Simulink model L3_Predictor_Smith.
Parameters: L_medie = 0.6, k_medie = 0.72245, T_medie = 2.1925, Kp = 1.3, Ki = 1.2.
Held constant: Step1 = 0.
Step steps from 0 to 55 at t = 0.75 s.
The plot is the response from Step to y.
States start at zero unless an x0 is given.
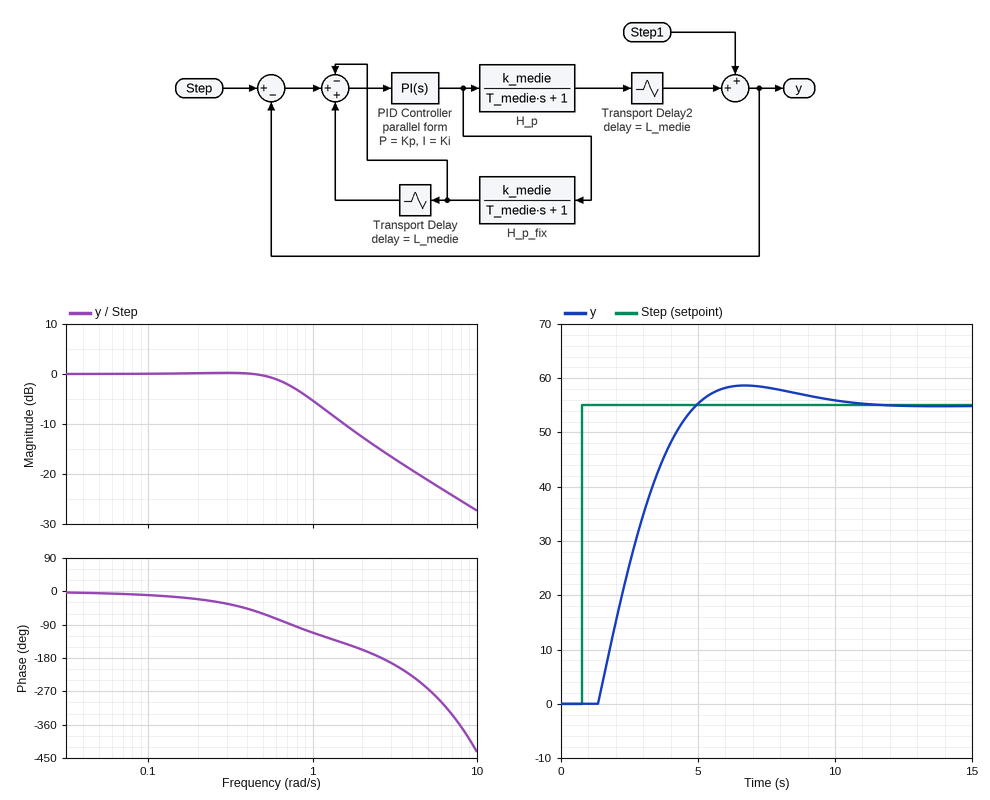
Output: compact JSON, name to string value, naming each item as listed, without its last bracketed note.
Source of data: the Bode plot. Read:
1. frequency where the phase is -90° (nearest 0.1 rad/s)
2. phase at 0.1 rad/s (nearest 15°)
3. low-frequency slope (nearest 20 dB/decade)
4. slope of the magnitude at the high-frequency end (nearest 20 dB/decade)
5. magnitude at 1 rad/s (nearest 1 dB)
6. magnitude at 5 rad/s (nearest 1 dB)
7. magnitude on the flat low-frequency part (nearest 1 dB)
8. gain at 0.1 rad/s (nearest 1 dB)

{"frequency where the phase is -90°": "0.7 rad/s", "phase at 0.1 rad/s": "-15°", "low-frequency slope": "0 dB/decade", "slope of the magnitude at the high-frequency end": "-20 dB/decade", "magnitude at 1 rad/s": "-5 dB", "magnitude at 5 rad/s": "-21 dB", "magnitude on the flat low-frequency part": "0 dB", "gain at 0.1 rad/s": "0 dB"}
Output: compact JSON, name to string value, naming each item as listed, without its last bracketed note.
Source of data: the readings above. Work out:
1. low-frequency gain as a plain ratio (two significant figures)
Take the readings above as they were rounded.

{"low-frequency gain as a plain ratio": "1.0"}
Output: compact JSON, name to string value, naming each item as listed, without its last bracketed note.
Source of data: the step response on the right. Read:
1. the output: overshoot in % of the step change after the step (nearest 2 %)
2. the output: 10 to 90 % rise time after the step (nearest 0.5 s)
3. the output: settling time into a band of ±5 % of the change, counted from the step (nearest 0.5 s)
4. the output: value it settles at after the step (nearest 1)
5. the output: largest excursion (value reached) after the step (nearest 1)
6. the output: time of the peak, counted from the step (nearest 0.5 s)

{"the output: overshoot in % of the step change after the step": "6 %", "the output: 10 to 90 % rise time after the step": "2.5 s", "the output: settling time into a band of ±5 % of the change, counted from the step": "7.5 s", "the output: value it settles at after the step": "55", "the output: largest excursion (value reached) after the step": "59", "the output: time of the peak, counted from the step": "6.0 s"}
